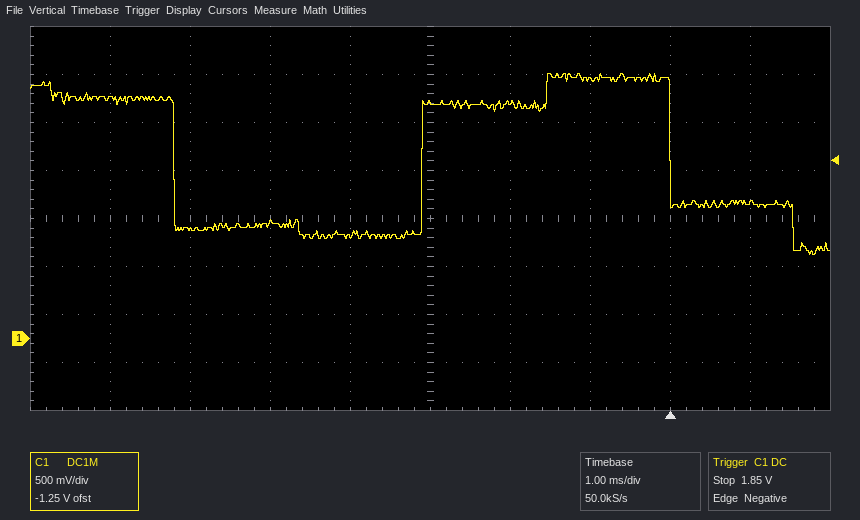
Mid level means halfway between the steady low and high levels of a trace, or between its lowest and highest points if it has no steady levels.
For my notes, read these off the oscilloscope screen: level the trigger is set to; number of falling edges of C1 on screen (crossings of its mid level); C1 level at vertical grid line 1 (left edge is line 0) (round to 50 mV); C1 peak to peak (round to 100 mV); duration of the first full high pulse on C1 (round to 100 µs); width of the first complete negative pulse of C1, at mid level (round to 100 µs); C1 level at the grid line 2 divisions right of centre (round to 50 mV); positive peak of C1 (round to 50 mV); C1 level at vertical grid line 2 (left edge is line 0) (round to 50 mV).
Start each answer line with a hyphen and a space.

- 1.85 V
- 2
- 2.50 V
- 1.90 V
- 3.1 ms
- 3.1 ms
- 2.70 V
- 2.75 V
- 1.15 V
